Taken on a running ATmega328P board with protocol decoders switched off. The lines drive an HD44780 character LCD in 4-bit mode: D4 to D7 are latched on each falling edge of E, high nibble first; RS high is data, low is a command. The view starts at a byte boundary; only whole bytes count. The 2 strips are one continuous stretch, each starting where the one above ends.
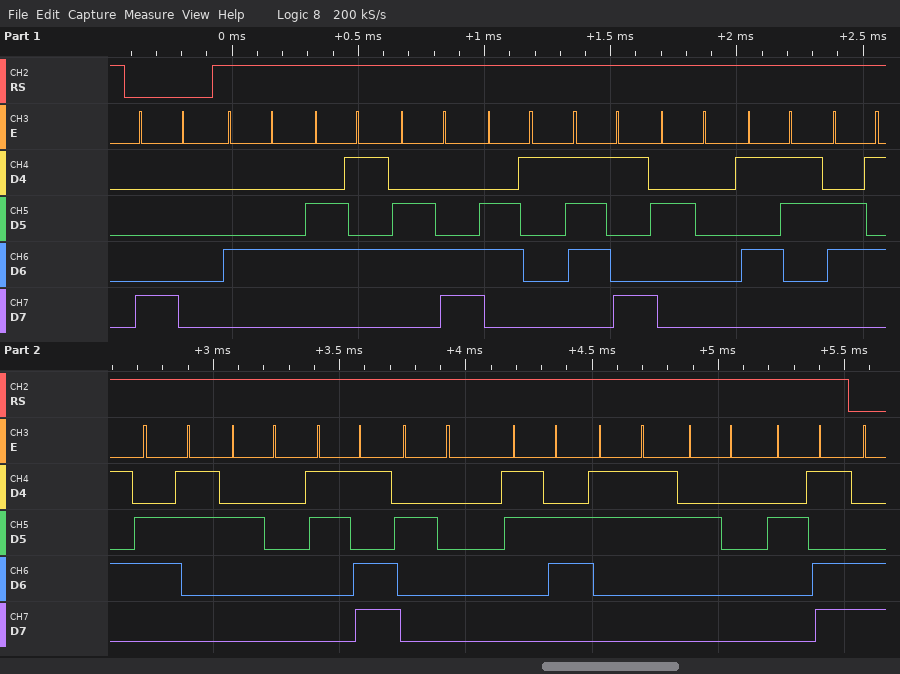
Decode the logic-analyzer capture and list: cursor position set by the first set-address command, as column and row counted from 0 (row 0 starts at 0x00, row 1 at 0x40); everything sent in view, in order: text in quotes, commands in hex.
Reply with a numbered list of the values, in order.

1. column 0, row 0
2. 0x80 "Delay Sec = 63 -"
